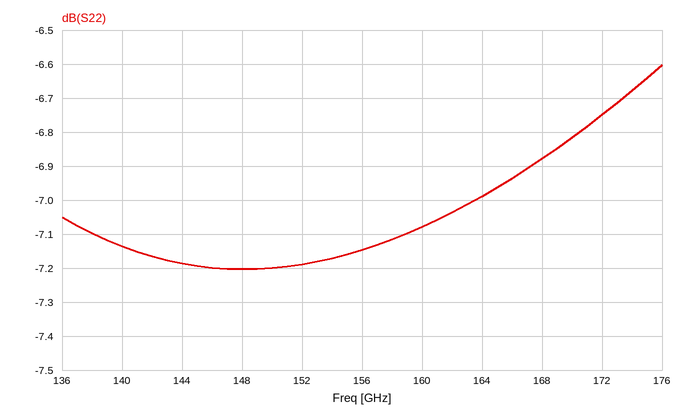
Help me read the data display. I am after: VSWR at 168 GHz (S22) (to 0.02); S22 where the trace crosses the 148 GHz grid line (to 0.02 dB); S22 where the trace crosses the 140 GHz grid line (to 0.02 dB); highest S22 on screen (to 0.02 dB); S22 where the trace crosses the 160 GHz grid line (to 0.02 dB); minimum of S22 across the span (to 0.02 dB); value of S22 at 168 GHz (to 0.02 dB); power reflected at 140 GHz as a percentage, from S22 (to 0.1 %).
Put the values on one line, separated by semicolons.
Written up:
2.66; -7.20 dB; -7.14 dB; -6.60 dB; -7.08 dB; -7.20 dB; -6.88 dB; 19.3 %
